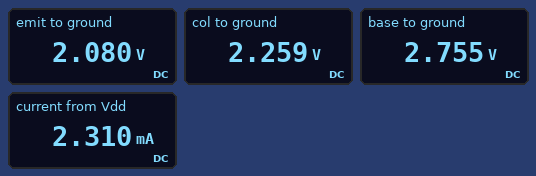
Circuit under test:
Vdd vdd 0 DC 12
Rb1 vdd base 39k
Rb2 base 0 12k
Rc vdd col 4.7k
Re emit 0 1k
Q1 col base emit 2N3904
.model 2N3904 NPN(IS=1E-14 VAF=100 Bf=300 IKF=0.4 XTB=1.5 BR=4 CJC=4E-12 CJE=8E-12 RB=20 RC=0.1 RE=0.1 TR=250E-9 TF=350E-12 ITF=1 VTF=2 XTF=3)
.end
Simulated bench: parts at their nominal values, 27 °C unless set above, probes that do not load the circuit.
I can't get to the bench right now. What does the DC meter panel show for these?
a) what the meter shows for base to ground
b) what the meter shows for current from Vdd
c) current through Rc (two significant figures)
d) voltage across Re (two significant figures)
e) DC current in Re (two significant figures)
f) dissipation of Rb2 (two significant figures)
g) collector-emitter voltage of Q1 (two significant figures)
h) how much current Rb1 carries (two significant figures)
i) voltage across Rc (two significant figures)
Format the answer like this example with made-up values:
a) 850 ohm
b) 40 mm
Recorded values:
a) 2.755 V
b) 2.310 mA
c) 2.1 mA
d) 2.1 V
e) 2.1 mA
f) 630 µW
g) 180 mV
h) 240 µA
i) 9.7 V
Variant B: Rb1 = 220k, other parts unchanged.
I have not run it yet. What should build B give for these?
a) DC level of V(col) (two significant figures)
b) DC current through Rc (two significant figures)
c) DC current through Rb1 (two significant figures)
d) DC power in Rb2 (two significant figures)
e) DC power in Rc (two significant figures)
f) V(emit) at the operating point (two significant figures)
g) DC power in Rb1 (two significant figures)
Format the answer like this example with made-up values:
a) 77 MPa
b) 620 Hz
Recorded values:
a) 12 V
b) 46 µA
c) 52 µA
d) 32 µW
e) 10 µW
f) 46 mV
g) 590 µW
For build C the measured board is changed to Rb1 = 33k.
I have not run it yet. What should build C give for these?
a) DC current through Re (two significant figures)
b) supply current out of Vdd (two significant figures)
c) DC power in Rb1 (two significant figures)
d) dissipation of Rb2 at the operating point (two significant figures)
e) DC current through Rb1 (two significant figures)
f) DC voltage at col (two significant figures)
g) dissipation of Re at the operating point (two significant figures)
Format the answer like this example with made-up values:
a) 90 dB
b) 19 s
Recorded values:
a) 2.1 mA
b) 2.4 mA
c) 2.6 mW
d) 660 µW
e) 280 µA
f) 2.2 V
g) 4.5 mW
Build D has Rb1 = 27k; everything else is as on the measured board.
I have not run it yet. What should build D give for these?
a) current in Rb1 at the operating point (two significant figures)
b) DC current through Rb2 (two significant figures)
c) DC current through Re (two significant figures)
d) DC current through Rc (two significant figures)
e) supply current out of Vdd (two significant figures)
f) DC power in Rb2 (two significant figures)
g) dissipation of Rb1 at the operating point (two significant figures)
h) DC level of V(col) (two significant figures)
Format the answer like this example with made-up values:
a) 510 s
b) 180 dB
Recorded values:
a) 340 µA
b) 240 µA
c) 2.2 mA
d) 2.1 mA
e) 2.4 mA
f) 680 µW
g) 3.1 mW
h) 2.2 V
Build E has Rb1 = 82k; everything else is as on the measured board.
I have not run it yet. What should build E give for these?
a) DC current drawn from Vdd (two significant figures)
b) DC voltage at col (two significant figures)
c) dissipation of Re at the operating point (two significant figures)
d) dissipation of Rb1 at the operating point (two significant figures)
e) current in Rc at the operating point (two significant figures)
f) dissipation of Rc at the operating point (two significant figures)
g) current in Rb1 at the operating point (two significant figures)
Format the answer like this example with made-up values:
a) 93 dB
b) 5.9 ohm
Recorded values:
a) 980 µA
b) 8.0 V
c) 730 µW
d) 1.3 mW
e) 850 µA
f) 3.4 mW
g) 130 µA
